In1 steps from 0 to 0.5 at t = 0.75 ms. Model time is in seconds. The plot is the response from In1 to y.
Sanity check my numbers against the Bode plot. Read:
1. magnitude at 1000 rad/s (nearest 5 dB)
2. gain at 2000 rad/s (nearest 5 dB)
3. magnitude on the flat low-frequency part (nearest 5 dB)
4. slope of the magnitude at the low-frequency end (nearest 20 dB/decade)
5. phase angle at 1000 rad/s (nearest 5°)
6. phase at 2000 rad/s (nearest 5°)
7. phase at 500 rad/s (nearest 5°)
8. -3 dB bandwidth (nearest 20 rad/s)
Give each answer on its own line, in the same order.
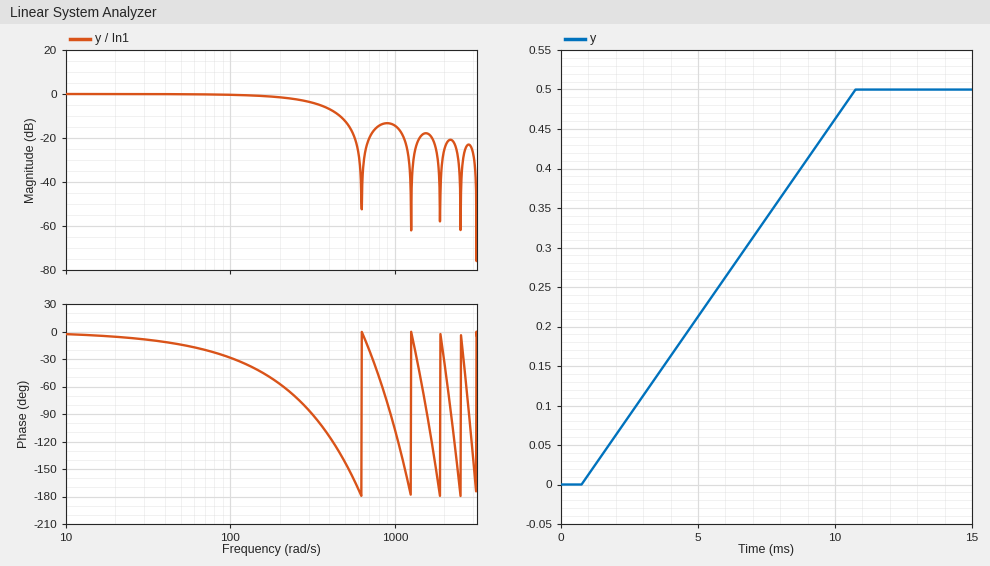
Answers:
-15 dB
-25 dB
0 dB
0 dB/decade
-105°
-35°
-145°
280 rad/s
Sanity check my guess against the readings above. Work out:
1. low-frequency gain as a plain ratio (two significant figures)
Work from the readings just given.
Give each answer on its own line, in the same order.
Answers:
1.0
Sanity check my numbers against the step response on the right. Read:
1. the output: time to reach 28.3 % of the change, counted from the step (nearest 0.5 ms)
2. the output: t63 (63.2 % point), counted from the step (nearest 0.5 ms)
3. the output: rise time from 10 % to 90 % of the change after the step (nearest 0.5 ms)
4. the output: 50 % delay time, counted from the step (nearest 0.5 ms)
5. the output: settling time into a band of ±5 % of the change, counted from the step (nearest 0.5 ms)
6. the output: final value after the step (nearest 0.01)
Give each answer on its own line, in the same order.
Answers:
3.0 ms
6.5 ms
8.0 ms
5.0 ms
9.5 ms
0.50
